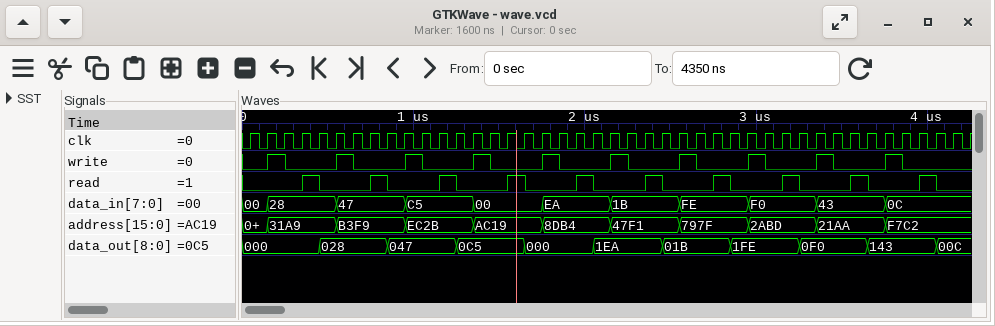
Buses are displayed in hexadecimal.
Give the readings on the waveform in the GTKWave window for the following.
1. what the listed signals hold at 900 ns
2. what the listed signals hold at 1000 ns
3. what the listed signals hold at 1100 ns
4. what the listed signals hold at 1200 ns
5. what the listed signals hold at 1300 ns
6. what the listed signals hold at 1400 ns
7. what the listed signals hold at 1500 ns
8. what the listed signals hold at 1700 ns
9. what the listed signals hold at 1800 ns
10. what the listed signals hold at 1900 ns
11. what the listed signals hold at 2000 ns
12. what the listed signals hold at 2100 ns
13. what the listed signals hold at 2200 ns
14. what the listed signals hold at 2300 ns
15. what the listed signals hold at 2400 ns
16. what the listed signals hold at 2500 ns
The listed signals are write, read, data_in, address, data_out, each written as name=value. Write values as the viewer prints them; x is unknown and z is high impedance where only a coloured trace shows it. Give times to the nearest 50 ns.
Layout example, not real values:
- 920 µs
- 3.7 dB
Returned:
- write=0, read=0, data_in=47, address=B3F9, data_out=047
- write=1, read=0, data_in=C5, address=EC2B, data_out=047
- write=0, read=0, data_in=C5, address=EC2B, data_out=047
- write=0, read=1, data_in=C5, address=EC2B, data_out=047
- write=0, read=0, data_in=C5, address=EC2B, data_out=0C5
- write=1, read=0, data_in=00, address=AC19, data_out=0C5
- write=0, read=0, data_in=00, address=AC19, data_out=0C5
- write=0, read=0, data_in=00, address=AC19, data_out=000
- write=1, read=0, data_in=EA, address=8DB4, data_out=000
- write=0, read=0, data_in=EA, address=8DB4, data_out=000
- write=0, read=1, data_in=EA, address=8DB4, data_out=000
- write=0, read=0, data_in=EA, address=8DB4, data_out=1EA
- write=1, read=0, data_in=1B, address=47F1, data_out=1EA
- write=0, read=0, data_in=1B, address=47F1, data_out=1EA
- write=0, read=1, data_in=1B, address=47F1, data_out=1EA
- write=0, read=0, data_in=1B, address=47F1, data_out=01B
